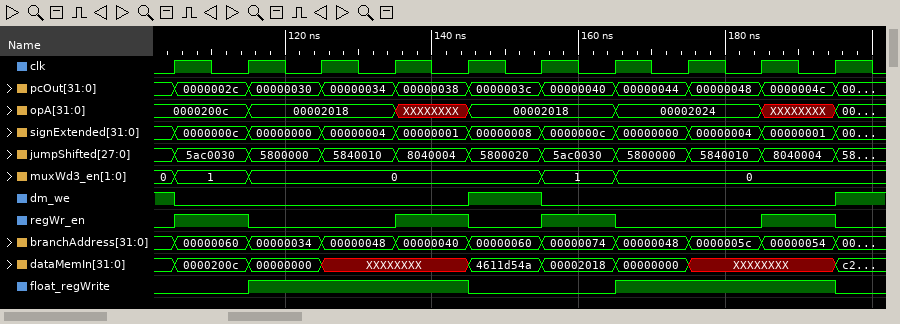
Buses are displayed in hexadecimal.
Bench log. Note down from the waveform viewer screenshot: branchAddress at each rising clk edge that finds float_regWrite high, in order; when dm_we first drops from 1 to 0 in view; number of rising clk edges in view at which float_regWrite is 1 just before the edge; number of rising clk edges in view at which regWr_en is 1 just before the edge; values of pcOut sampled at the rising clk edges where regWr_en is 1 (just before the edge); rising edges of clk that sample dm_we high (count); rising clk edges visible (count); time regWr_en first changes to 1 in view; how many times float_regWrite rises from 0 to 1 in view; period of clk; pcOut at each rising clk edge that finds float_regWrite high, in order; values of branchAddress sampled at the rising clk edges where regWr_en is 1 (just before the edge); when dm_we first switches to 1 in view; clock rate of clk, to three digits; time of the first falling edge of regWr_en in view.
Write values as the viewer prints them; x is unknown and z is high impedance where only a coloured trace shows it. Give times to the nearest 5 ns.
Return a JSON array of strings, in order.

["00000034, 00000048, 00000040, 00000048, 0000005c, 00000054", "105 ns", "6", "4", "0000002c, 00000038, 00000040, 0000004c", "2", "10", "105 ns", "2", "10 ns", "00000030, 00000034, 00000038, 00000044, 00000048, 0000004c", "00000060, 00000040, 00000074, 00000054", "145 ns", "100 MHz", "115 ns"]
